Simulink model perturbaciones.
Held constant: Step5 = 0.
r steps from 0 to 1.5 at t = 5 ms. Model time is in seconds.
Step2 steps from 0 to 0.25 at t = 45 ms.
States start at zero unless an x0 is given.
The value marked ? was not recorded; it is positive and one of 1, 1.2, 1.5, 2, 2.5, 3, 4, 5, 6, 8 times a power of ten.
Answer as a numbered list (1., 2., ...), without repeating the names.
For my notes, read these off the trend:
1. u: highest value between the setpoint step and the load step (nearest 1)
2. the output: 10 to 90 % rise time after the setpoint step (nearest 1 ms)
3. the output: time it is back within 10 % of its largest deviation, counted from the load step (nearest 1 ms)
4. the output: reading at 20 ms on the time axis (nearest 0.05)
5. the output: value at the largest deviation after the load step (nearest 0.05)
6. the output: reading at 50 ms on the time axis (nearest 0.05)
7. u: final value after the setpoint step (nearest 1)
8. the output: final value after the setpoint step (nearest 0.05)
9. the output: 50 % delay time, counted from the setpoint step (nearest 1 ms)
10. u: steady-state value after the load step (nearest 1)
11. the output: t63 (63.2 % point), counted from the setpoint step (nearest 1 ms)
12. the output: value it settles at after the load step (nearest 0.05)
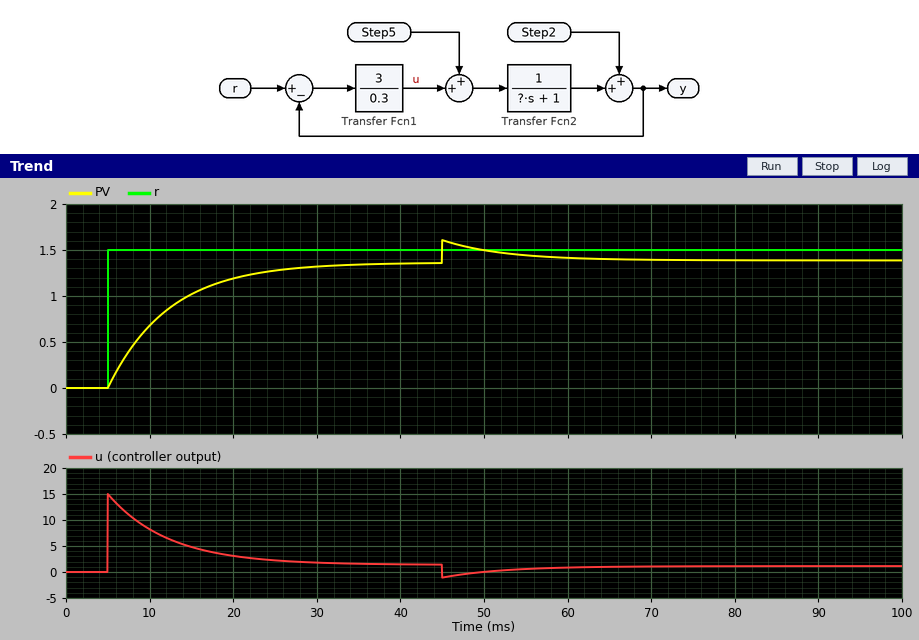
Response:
1. 15
2. 16 ms
3. 16 ms
4. 1.20
5. 1.60
6. 1.50
7. 1
8. 1.35
9. 5 ms
10. 1
11. 7 ms
12. 1.40
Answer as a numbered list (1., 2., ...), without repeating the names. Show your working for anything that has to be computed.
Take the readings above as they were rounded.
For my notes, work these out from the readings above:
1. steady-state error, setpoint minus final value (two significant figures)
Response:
1. 1.5 - 1.35 = 0.15
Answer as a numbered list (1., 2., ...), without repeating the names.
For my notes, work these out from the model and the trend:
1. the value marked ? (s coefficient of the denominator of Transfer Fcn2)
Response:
1. 0.08
